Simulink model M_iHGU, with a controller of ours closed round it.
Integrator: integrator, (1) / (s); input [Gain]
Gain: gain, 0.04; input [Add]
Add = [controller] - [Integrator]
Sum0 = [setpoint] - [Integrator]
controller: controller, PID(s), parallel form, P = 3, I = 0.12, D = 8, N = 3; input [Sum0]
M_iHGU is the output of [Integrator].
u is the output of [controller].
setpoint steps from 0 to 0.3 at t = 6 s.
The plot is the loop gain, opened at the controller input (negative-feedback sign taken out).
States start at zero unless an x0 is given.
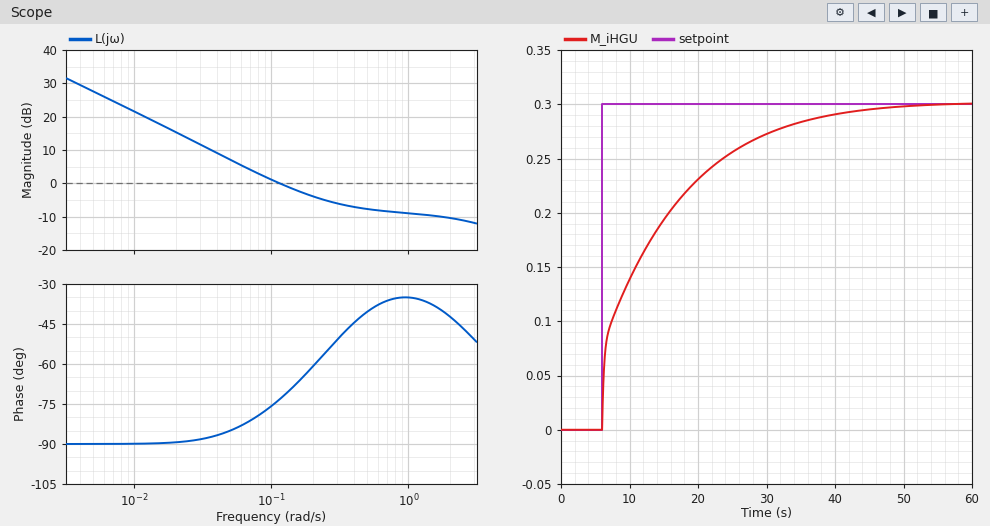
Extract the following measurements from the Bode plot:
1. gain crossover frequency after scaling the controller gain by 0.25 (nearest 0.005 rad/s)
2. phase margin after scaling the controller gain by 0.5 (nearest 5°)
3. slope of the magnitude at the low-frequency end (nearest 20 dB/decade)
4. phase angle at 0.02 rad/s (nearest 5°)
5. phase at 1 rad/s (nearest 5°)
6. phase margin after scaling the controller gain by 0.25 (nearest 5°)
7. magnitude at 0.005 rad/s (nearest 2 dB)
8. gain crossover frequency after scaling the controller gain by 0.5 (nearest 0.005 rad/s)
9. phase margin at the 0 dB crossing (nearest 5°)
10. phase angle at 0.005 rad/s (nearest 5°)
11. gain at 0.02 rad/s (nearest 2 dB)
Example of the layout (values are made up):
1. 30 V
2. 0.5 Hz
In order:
1. 0.030 rad/s
2. 95°
3. -20 dB/decade
4. -90°
5. -35°
6. 90°
7. 28 dB
8. 0.055 rad/s
9. 105°
10. -90°
11. 16 dB
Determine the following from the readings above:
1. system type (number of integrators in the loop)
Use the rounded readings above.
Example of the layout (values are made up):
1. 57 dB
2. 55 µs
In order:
1. 1
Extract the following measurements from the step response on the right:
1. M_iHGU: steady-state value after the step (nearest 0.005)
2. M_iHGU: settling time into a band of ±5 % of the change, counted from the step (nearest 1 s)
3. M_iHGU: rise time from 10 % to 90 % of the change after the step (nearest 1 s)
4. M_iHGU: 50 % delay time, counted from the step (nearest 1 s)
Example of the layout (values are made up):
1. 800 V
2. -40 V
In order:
1. 0.300
2. 30 s
3. 23 s
4. 5 s
